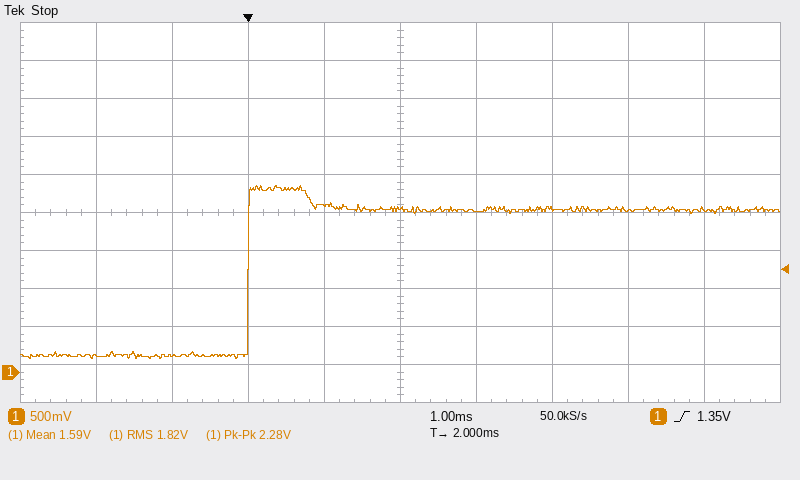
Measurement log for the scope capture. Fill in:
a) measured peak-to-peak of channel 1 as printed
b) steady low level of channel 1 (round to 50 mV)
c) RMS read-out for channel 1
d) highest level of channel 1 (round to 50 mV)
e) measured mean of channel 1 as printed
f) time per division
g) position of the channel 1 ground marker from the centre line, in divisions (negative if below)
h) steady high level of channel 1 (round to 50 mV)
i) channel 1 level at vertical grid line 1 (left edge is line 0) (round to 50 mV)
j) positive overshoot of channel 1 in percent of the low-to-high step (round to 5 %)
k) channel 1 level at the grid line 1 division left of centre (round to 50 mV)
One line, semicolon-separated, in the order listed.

2.28 V; 200 mV; 1.82 V; 2.45 V; 1.59 V; 1 ms; -4.2 div; 2.15 V; 200 mV; 15 %; 2.20 V
